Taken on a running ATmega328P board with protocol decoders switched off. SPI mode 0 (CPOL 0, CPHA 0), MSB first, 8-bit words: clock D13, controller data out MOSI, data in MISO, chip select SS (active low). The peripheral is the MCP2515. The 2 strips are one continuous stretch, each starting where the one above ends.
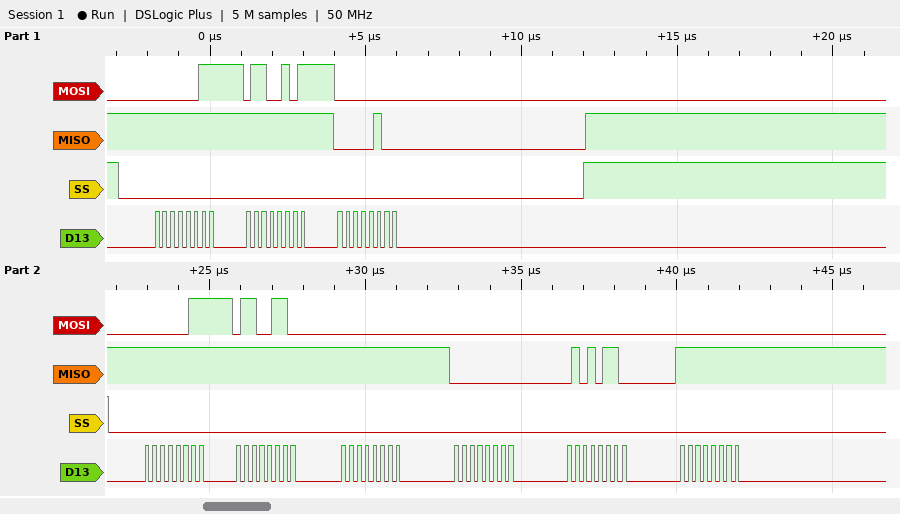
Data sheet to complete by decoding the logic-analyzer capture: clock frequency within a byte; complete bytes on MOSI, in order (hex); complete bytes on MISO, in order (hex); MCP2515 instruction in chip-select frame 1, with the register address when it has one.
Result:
4 MHz
03 65 00 03 66 00 00 00 00
FF FF 04 FF FF FF 00 56 FF
READ 0x65
